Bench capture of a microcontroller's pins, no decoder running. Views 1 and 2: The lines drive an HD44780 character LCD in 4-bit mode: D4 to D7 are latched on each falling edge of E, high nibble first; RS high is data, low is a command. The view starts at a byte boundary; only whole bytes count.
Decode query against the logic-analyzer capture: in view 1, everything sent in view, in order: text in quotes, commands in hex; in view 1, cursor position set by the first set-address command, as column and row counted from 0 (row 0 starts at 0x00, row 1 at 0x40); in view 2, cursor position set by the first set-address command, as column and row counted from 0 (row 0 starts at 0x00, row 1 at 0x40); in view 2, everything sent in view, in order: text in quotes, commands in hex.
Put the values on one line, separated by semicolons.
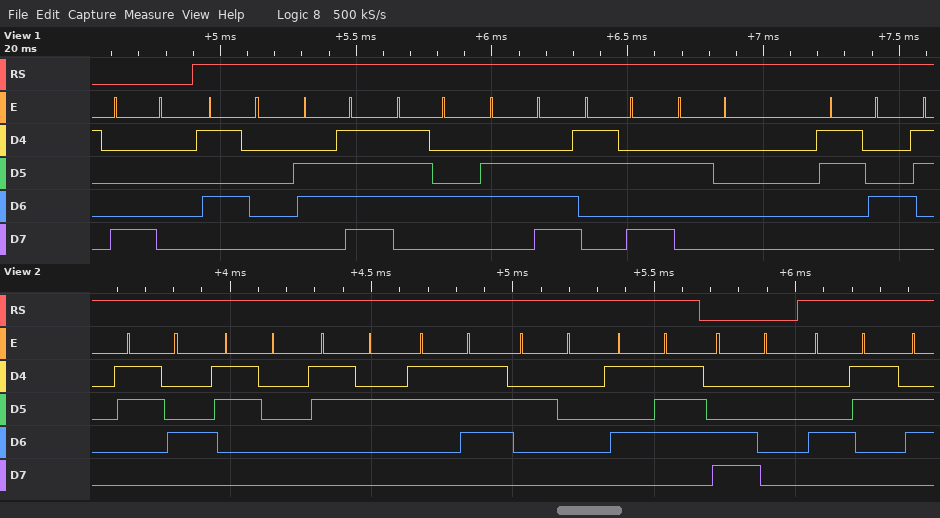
0x80 "Potn: 4"; column 0, row 0; column 0, row 1; "4027 W" 0xC0 "C"
